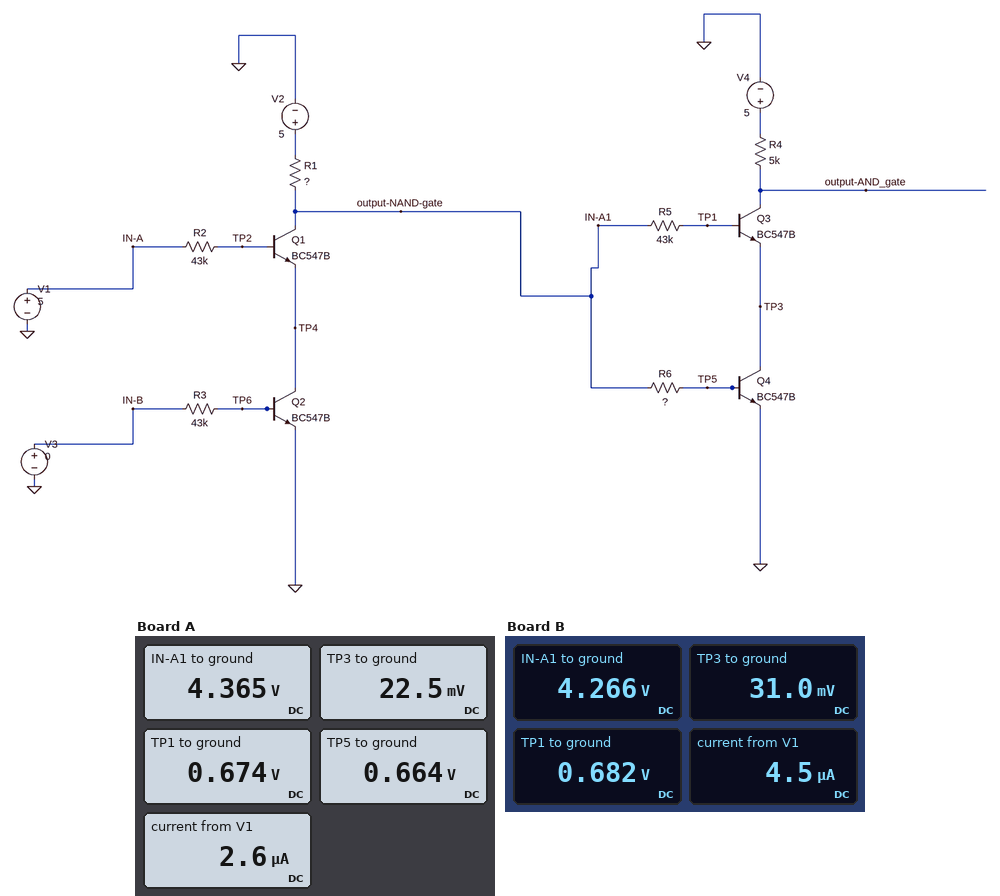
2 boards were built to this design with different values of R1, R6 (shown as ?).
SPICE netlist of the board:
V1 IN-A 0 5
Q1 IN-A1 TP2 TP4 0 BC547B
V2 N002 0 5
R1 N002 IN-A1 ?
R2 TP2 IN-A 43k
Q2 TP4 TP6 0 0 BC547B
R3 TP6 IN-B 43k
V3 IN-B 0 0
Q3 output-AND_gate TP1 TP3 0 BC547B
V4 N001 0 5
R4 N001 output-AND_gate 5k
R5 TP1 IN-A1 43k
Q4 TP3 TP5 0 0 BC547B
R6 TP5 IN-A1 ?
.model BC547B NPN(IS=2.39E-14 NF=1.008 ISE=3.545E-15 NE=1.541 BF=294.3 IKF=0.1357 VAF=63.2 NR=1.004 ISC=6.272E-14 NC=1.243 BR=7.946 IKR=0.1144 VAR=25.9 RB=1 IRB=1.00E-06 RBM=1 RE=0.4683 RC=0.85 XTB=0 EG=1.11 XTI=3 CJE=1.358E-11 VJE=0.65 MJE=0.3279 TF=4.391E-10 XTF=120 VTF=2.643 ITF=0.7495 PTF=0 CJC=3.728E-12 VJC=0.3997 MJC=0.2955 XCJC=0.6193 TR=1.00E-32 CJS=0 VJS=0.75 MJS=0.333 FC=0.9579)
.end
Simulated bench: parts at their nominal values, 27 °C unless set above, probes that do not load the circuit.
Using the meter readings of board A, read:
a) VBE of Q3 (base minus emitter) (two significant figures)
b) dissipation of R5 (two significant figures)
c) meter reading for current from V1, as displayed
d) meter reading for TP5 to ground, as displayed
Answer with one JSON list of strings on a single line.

["650 mV", "320 µW", "2.6 µA", "0.664 V"]
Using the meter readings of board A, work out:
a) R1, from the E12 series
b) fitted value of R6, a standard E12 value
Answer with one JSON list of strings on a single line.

["2.2 kΩ", "18 kΩ"]
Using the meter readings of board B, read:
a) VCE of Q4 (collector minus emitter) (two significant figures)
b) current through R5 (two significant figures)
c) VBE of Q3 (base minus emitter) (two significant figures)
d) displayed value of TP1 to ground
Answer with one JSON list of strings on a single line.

["31 mV", "83 µA", "650 mV", "0.682 V"]
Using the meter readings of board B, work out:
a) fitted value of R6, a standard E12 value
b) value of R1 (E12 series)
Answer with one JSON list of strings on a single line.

["33 kΩ", "3.9 kΩ"]
